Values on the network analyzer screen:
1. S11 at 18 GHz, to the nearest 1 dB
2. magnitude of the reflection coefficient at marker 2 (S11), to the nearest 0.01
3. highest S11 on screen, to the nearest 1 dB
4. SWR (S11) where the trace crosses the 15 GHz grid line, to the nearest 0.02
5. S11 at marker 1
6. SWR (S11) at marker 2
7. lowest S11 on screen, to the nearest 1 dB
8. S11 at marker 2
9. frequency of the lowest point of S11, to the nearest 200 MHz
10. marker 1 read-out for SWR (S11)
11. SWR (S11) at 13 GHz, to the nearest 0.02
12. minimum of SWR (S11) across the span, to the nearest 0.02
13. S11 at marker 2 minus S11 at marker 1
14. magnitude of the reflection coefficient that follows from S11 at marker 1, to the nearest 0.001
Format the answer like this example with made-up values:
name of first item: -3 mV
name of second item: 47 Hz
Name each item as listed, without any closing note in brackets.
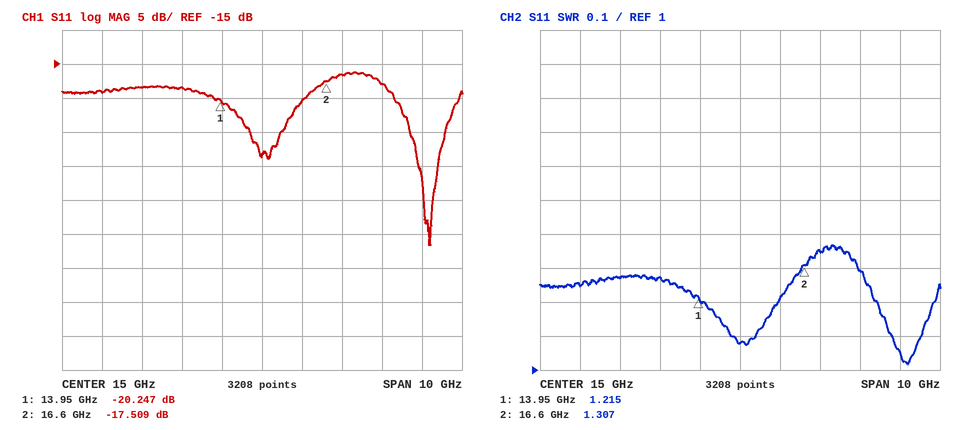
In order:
S11 at 18 GHz, to the nearest 1 dB: -18 dB
magnitude of the reflection coefficient at marker 2 (S11), to the nearest 0.01: 0.13
highest S11 on screen, to the nearest 1 dB: -16 dB
SWR (S11) where the trace crosses the 15 GHz grid line, to the nearest 0.02: 1.08
S11 at marker 1: -20.247 dB
SWR (S11) at marker 2: 1.307
lowest S11 on screen, to the nearest 1 dB: -42 dB
S11 at marker 2: -17.509 dB
frequency of the lowest point of S11, to the nearest 200 MHz: 19.2 GHz
marker 1 read-out for SWR: 1.215
SWR (S11) at 13 GHz, to the nearest 0.02: 1.28
minimum of SWR (S11) across the span, to the nearest 0.02: 1.02
S11 at marker 2 minus S11 at marker 1: 2.738 dB
magnitude of the reflection coefficient that follows from S11 at marker 1, to the nearest 0.001: 0.097
